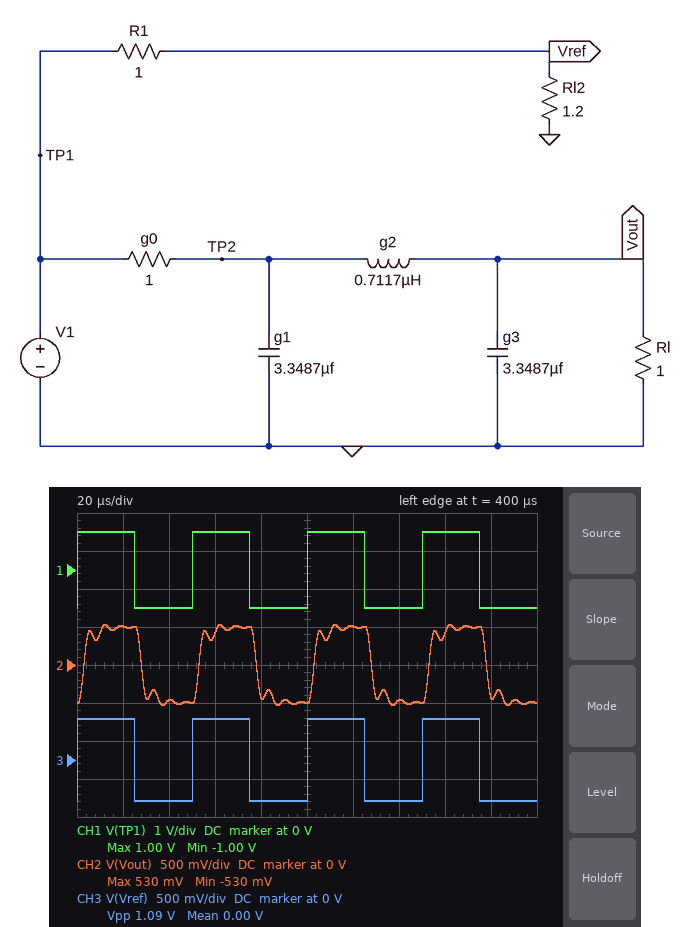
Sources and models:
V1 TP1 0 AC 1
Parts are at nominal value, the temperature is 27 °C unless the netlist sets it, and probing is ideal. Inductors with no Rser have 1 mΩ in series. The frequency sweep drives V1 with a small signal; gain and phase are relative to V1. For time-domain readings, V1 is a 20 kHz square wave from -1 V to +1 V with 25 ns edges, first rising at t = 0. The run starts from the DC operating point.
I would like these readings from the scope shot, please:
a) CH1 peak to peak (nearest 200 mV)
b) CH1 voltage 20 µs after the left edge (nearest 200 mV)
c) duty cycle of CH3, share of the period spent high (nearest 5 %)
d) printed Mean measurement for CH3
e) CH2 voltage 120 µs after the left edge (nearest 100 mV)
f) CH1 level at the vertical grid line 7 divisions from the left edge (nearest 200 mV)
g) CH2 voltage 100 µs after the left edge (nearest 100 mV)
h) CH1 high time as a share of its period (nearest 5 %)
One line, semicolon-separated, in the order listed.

2.0 V; 1.0 V; 50 %; 0.00 V; 500 mV; -1.0 V; -500 mV; 50 %
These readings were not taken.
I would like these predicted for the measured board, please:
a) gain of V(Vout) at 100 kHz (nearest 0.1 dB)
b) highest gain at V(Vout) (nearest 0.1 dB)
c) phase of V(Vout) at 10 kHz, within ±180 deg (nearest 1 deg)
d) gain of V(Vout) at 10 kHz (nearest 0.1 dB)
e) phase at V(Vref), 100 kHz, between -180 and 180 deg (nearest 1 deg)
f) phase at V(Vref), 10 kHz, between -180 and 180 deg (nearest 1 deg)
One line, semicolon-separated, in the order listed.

-8.6 dB; -6.0 dB; -13 deg; -6.2 dB; 0 deg; 0 deg
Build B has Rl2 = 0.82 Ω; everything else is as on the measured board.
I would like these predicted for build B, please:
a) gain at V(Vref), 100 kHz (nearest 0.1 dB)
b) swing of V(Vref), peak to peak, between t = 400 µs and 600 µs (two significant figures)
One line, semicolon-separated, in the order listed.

-6.9 dB; 900 mV
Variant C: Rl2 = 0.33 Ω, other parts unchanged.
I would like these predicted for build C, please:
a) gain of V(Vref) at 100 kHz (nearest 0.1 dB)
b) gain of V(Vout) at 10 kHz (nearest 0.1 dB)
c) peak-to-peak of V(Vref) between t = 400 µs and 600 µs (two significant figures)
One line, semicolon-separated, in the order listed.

-12.1 dB; -6.2 dB; 500 mV
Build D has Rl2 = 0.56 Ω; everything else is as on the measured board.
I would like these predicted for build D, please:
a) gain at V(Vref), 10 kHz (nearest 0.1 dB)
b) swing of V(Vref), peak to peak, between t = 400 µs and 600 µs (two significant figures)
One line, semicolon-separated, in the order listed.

-8.9 dB; 720 mV
